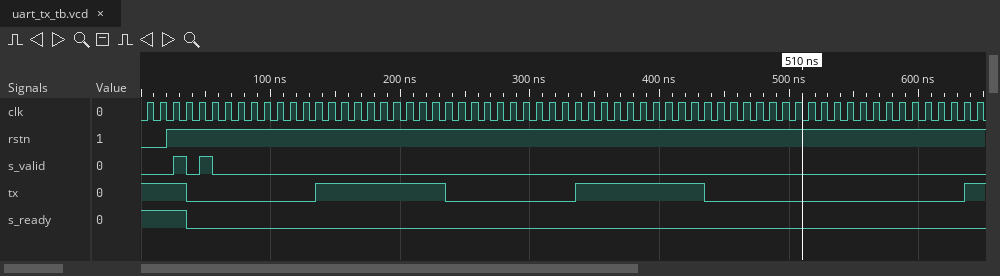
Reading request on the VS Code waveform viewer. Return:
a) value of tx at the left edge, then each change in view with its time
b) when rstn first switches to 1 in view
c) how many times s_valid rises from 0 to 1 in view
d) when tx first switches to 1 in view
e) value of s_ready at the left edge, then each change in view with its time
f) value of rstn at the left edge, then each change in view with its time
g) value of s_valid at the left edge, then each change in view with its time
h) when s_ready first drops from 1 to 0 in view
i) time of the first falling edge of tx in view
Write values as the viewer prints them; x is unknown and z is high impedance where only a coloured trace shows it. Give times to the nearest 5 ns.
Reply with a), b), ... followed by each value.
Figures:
a) 1, 0 at 35 ns, 1 at 135 ns, 0 at 235 ns, 1 at 335 ns, 0 at 435 ns, 1 at 635 ns
b) 20 ns
c) 2
d) 135 ns
e) 1, 0 at 35 ns
f) 0, 1 at 20 ns
g) 0, 1 at 25 ns, 0 at 35 ns, 1 at 45 ns, 0 at 55 ns
h) 35 ns
i) 35 ns
